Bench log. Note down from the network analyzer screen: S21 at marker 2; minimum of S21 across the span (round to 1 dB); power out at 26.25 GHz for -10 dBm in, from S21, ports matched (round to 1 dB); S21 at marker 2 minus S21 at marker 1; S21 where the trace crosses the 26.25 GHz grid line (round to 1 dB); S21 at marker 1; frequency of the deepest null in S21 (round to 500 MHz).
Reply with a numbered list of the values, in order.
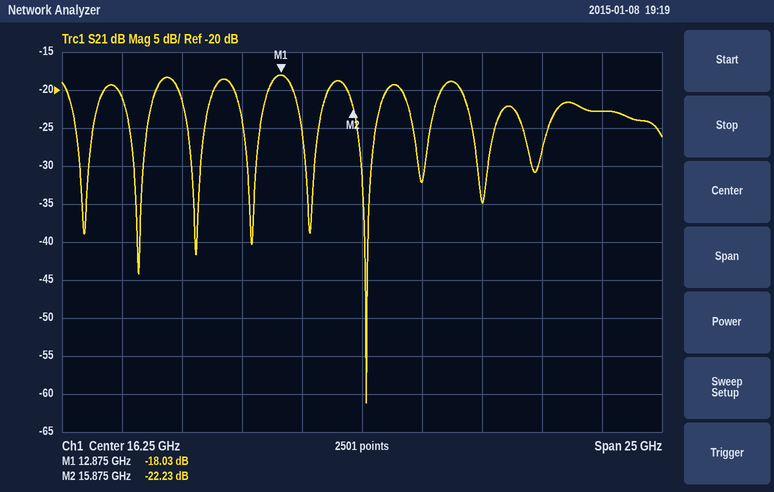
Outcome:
1. -22.23 dB
2. -61 dB
3. -33 dBm
4. -4.20 dB
5. -23 dB
6. -18.03 dB
7. 16.5 GHz
